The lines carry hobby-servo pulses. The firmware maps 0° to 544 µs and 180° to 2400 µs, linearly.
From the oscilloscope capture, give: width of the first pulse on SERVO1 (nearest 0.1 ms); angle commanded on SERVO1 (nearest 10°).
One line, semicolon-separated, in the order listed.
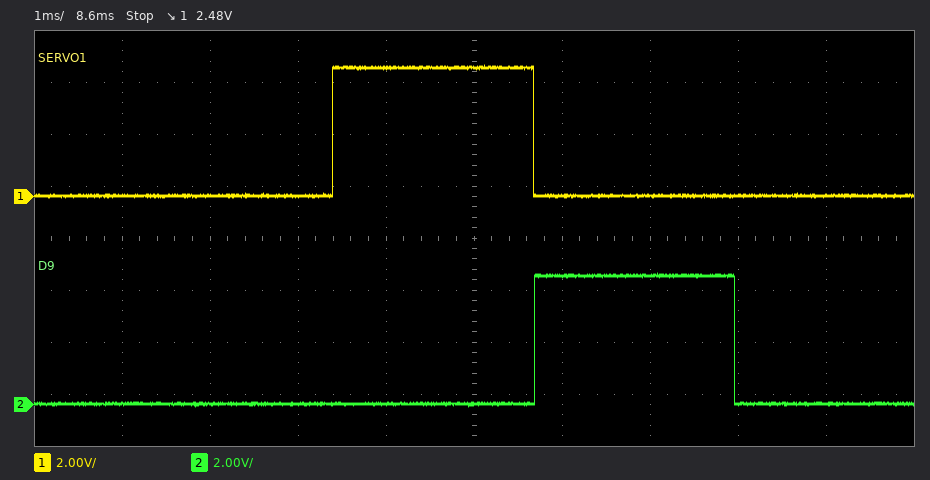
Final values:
2.3 ms; 170°
